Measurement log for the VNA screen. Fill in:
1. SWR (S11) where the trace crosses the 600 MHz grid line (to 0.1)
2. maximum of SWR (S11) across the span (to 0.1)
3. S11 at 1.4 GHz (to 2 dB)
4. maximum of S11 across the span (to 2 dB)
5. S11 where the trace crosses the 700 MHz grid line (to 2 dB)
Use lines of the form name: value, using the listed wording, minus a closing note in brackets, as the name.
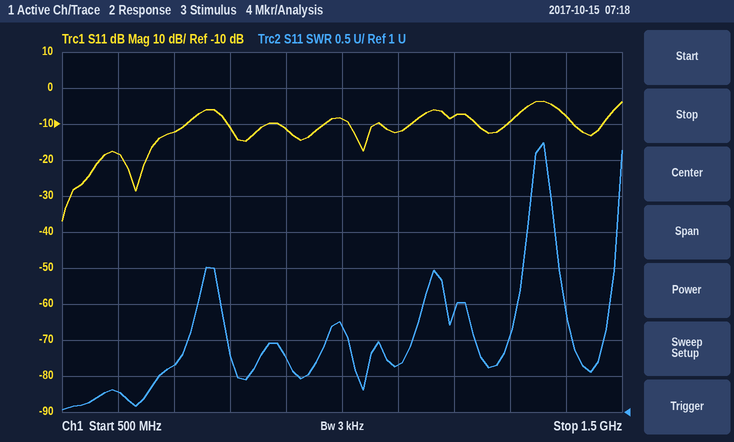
SWR (S11) where the trace crosses the 600 MHz grid line: 1.3
maximum of SWR (S11) across the span: 4.7
S11 at 1.4 GHz: -8 dB
maximum of S11 across the span: -4 dB
S11 where the trace crosses the 700 MHz grid line: -12 dB
